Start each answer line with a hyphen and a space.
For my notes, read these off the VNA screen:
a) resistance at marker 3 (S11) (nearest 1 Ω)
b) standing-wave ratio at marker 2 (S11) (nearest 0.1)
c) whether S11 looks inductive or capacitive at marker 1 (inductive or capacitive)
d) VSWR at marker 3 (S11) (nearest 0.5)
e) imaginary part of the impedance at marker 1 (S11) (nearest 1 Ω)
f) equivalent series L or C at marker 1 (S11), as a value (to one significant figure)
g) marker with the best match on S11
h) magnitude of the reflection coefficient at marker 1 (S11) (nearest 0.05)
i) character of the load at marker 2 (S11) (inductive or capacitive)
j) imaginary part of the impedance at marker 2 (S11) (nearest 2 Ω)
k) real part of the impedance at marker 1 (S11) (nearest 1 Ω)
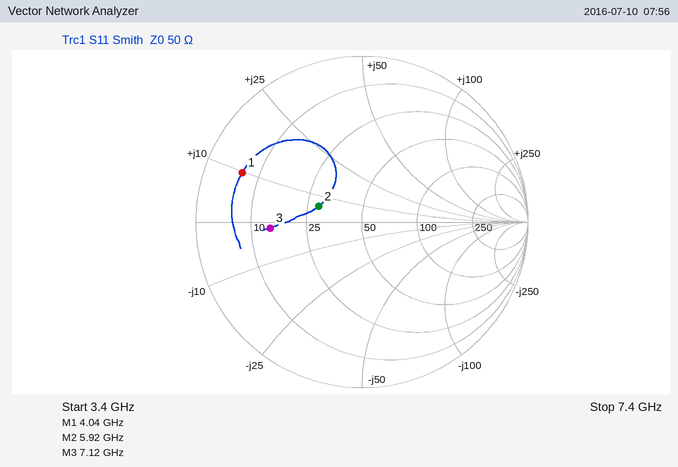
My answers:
- 14 Ω
- 1.8
- inductive
- 3.5
- +10 Ω
- 400 pH
- marker 2
- 0.80
- inductive
- +6 Ω
- 6 Ω
